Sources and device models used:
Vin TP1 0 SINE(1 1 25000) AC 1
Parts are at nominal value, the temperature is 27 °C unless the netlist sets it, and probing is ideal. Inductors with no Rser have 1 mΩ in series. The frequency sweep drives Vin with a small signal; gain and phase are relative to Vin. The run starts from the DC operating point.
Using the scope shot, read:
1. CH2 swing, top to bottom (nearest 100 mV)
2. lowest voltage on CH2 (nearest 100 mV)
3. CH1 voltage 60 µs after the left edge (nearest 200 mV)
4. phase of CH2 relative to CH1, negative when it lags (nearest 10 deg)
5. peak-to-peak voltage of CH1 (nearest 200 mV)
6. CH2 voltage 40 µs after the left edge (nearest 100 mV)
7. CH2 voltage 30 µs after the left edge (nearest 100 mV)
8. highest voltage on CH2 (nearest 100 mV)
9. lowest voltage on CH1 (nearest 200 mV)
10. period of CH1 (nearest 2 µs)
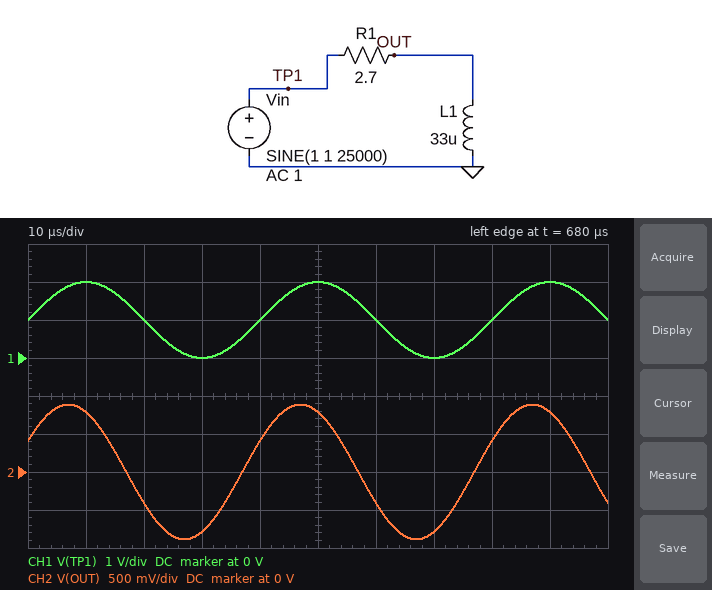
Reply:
1.8 V
-900 mV
1.0 V
30 deg
2.0 V
400 mV
-800 mV
900 mV
0 V
40 µs
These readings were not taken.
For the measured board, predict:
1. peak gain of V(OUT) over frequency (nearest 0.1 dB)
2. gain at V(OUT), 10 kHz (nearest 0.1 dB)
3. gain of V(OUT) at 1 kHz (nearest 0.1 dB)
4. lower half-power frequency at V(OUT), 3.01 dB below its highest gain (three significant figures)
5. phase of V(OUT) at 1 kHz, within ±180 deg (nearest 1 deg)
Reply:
0 dB
-4.3 dB
-22.3 dB
13.0 kHz
85 deg
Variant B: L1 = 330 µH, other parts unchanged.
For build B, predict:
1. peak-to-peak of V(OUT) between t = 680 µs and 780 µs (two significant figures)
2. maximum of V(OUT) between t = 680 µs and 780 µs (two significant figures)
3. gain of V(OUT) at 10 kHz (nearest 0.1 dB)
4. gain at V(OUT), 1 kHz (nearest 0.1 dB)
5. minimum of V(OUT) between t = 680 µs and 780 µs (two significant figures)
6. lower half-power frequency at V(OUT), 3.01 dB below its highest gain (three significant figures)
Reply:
2.0 V
1.0 V
-0.1 dB
-4.3 dB
-1.0 V
1.30 kHz
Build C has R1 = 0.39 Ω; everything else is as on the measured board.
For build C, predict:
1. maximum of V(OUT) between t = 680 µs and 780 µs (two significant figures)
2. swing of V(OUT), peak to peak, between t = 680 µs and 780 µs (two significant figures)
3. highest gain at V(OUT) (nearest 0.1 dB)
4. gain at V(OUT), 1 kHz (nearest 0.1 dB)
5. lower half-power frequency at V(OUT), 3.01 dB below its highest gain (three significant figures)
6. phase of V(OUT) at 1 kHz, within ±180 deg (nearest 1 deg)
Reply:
1.0 V
2.0 V
0 dB
-6.6 dB
1.89 kHz
62 deg
